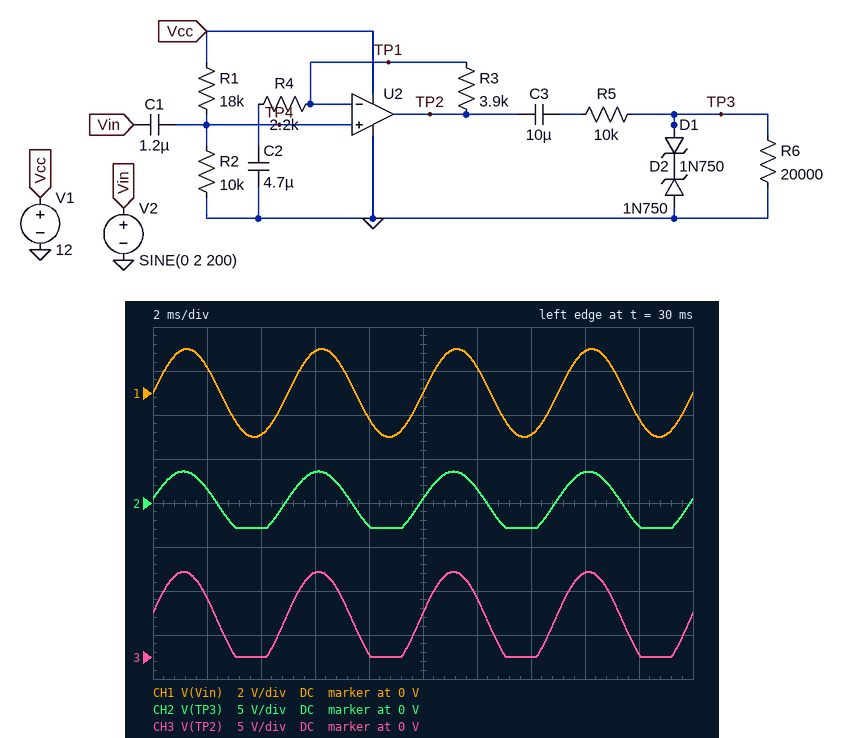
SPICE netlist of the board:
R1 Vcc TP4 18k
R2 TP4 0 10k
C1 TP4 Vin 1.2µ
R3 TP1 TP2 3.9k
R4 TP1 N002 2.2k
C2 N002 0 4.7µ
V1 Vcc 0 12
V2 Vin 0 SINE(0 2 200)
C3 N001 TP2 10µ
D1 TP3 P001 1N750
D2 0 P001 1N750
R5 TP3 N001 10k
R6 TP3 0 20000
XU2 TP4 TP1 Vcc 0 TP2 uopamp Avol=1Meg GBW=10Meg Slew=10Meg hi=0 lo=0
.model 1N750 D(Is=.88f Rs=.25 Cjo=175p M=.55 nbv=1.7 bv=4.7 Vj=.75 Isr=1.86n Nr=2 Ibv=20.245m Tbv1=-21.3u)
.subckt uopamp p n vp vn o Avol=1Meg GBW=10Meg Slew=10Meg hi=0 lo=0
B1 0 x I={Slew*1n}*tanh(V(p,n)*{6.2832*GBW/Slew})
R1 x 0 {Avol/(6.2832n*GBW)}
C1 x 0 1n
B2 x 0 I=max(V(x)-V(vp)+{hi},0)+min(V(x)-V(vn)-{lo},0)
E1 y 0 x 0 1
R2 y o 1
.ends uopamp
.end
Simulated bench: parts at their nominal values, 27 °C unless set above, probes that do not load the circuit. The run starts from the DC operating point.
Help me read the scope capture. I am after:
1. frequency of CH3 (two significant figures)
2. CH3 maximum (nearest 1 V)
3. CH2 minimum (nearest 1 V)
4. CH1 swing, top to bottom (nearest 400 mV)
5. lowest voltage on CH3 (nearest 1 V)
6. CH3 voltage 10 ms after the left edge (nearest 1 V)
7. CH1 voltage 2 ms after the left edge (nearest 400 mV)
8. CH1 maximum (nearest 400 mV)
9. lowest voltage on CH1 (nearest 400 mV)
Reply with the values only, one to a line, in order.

200 Hz
10 V
-3 V
4.0 V
0 V
5 V
1.2 V
2.0 V
-2.0 V
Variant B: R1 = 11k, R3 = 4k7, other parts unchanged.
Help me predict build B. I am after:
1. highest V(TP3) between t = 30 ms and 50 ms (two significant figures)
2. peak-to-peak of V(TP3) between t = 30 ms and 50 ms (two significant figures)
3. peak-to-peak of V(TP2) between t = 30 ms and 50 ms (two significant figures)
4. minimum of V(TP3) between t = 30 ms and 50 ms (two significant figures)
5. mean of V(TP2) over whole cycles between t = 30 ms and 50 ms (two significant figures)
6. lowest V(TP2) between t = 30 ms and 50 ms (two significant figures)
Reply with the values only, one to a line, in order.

4.1 V
7.9 V
12 V
-3.8 V
5.7 V
-6.7 mV
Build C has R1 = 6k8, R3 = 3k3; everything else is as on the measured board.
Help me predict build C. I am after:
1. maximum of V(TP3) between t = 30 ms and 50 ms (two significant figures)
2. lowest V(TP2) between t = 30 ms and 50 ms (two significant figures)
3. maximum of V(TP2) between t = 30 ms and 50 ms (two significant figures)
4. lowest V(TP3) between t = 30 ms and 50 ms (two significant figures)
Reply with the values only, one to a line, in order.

3.2 V
2.2 V
12 V
-3.3 V
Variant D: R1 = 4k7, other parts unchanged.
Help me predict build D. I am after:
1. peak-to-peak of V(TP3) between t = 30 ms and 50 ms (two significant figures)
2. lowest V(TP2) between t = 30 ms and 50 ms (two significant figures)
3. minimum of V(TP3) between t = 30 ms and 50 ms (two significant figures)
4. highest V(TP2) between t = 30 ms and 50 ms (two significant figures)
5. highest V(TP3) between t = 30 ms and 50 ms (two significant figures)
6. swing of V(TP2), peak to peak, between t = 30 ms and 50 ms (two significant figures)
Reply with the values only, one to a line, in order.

6.1 V
2.9 V
-3.5 V
12 V
2.6 V
9.1 V
